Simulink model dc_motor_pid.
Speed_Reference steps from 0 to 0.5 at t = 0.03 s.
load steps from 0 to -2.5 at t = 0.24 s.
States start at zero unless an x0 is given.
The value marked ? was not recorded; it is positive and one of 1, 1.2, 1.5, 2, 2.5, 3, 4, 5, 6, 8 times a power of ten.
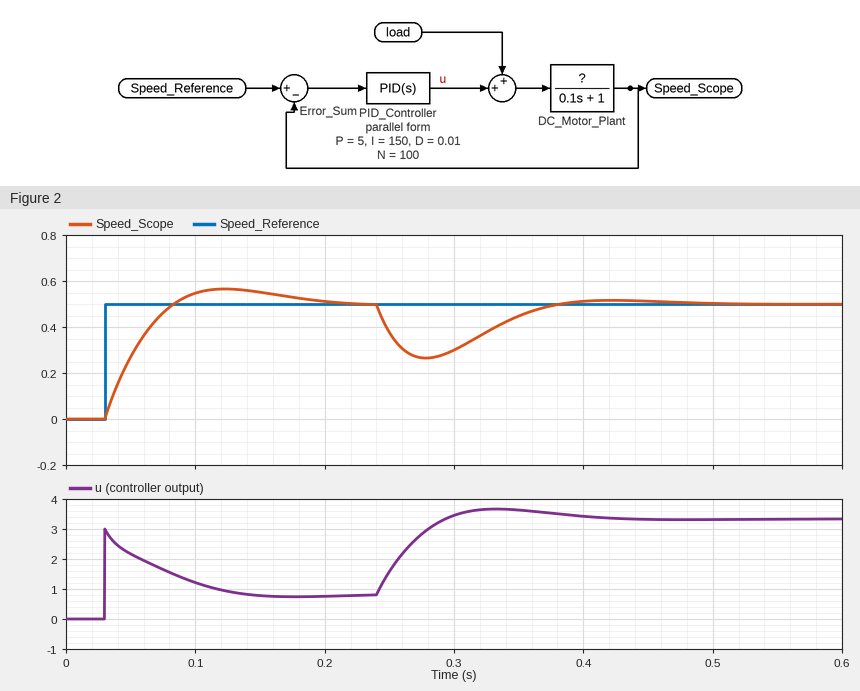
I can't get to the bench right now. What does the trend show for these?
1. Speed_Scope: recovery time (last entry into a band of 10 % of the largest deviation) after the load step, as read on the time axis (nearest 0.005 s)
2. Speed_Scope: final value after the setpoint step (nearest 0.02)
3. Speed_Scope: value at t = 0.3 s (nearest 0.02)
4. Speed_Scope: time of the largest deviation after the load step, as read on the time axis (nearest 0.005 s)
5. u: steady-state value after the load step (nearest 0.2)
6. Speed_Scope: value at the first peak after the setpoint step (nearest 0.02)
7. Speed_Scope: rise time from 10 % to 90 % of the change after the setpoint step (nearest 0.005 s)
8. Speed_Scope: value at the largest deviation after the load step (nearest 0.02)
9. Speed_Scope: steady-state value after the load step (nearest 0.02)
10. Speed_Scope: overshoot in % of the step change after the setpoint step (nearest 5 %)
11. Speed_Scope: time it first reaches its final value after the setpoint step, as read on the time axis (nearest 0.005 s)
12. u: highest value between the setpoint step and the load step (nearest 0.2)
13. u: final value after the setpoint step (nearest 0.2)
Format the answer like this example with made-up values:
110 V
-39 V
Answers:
0.365 s
0.50
0.30
0.280 s
3.4
0.56
0.040 s
0.26
0.50
15 %
0.085 s
3.0
0.8
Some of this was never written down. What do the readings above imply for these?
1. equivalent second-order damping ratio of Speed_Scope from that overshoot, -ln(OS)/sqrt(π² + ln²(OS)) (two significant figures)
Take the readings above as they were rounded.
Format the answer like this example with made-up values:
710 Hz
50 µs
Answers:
0.52
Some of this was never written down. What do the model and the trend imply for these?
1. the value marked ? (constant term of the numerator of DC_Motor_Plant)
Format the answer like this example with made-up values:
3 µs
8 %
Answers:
0.6
